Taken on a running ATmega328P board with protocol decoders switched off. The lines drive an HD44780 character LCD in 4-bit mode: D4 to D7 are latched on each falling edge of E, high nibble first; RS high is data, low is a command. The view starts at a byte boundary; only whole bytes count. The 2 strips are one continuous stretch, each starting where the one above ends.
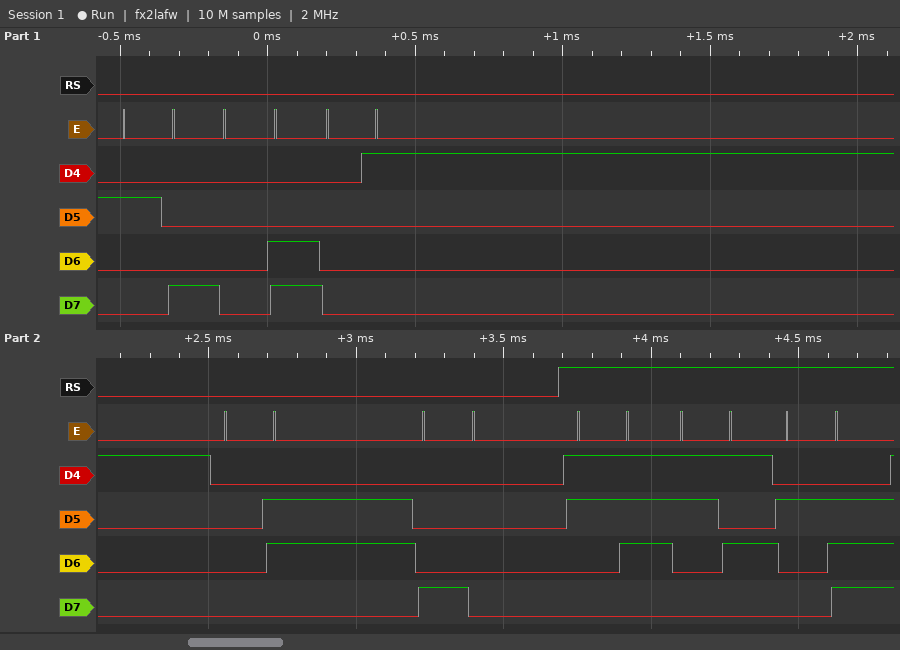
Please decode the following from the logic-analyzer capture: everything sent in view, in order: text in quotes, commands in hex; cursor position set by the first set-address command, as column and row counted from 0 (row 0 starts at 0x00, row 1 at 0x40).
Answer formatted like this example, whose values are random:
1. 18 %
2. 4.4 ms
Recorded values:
1. 0x28 0x0C 0x01 0x06 0x80 "75."
2. column 0, row 0
